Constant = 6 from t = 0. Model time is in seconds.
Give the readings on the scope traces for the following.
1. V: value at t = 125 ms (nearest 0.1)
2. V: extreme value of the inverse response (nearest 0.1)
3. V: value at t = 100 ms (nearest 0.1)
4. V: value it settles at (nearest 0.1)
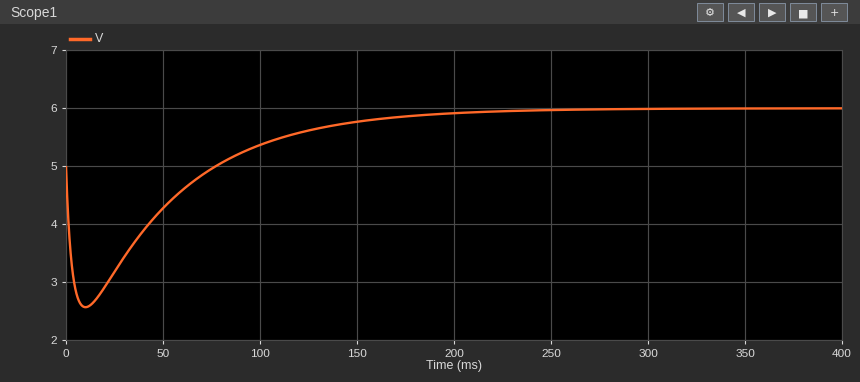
5.6
2.6
5.4
6.0
